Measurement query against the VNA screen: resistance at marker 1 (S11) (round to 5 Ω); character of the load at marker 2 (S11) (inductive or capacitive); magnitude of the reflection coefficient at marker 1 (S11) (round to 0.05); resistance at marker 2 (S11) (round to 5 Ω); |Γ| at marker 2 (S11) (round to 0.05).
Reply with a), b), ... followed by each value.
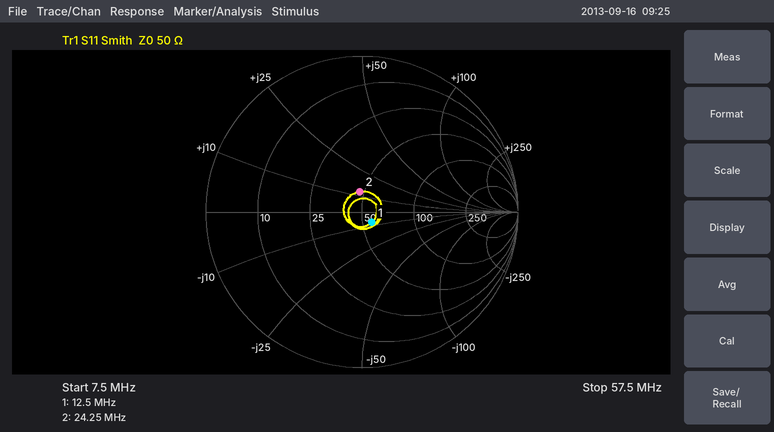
a) 55 Ω
b) inductive
c) 0.10
d) 45 Ω
e) 0.15
